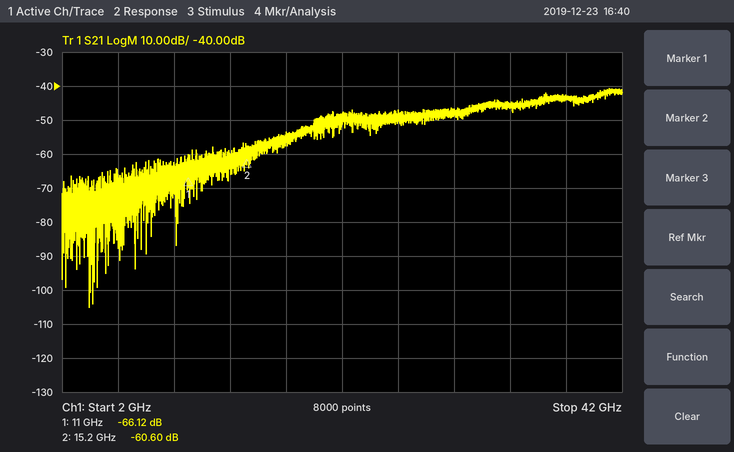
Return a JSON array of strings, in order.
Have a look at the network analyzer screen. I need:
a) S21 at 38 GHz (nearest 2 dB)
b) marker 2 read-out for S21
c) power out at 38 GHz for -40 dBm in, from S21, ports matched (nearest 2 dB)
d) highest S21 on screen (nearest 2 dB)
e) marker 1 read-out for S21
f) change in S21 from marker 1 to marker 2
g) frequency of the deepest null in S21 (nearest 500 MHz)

["-44 dB", "-60.60 dB", "-84 dBm", "-40 dB", "-66.12 dB", "5.52 dB", "4.0 GHz"]
